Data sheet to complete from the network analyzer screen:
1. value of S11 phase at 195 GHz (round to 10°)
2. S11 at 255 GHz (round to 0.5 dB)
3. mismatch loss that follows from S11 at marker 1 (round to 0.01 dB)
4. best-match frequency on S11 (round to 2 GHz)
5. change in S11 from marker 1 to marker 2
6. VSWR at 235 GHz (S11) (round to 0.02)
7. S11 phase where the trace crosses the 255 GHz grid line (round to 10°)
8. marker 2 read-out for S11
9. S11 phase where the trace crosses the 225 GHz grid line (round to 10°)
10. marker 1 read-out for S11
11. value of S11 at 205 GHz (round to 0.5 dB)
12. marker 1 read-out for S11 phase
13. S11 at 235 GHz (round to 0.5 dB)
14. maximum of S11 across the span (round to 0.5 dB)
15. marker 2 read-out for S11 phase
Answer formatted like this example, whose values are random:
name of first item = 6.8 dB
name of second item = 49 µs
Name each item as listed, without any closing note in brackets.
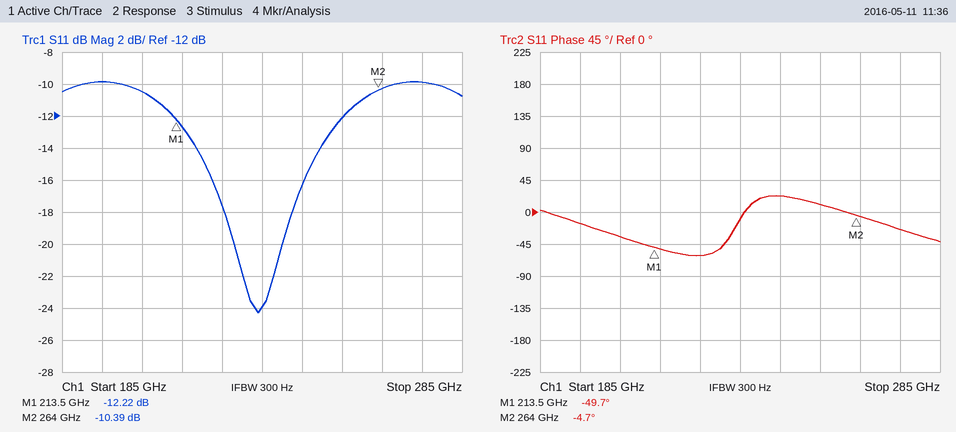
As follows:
value of S11 phase at 195 GHz = -20°
S11 at 255 GHz = -12.0 dB
mismatch loss that follows from S11 at marker 1 = 0.27 dB
best-match frequency on S11 = 234 GHz
change in S11 from marker 1 to marker 2 = 1.83 dB
VSWR at 235 GHz (S11) = 1.14
S11 phase where the trace crosses the 255 GHz grid line = 10°
marker 2 read-out for S11 = -10.39 dB
S11 phase where the trace crosses the 225 GHz grid line = -60°
marker 1 read-out for S11 = -12.22 dB
value of S11 at 205 GHz = -10.5 dB
marker 1 read-out for S11 phase = -49.7°
S11 at 235 GHz = -24.0 dB
maximum of S11 across the span = -10.0 dB
marker 2 read-out for S11 phase = -4.7°
